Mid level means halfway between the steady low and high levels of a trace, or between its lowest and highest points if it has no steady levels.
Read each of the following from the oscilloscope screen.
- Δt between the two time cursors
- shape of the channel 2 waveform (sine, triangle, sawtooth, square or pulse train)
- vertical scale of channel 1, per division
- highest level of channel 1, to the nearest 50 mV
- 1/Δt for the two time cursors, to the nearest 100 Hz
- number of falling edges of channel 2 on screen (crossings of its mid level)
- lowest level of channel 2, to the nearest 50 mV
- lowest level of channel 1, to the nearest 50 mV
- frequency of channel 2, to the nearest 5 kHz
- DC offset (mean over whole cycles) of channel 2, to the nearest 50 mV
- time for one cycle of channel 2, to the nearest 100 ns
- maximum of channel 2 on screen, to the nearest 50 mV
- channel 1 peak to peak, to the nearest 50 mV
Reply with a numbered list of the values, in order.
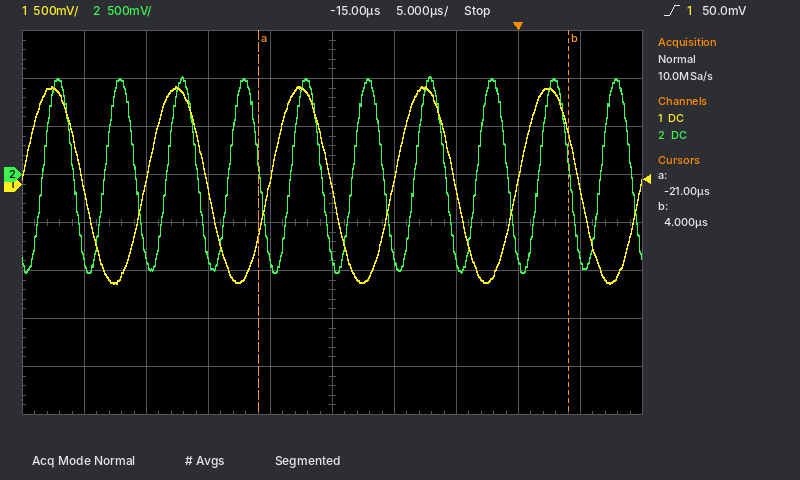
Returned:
1. 25.0 µs
2. sine
3. 500 mV
4. 1.00 V
5. 40.0 kHz
6. 10
7. -1.00 V
8. -1.05 V
9. 200 kHz
10. 0 mV
11. 5.0 µs
12. 1.00 V
13. 2.05 V
